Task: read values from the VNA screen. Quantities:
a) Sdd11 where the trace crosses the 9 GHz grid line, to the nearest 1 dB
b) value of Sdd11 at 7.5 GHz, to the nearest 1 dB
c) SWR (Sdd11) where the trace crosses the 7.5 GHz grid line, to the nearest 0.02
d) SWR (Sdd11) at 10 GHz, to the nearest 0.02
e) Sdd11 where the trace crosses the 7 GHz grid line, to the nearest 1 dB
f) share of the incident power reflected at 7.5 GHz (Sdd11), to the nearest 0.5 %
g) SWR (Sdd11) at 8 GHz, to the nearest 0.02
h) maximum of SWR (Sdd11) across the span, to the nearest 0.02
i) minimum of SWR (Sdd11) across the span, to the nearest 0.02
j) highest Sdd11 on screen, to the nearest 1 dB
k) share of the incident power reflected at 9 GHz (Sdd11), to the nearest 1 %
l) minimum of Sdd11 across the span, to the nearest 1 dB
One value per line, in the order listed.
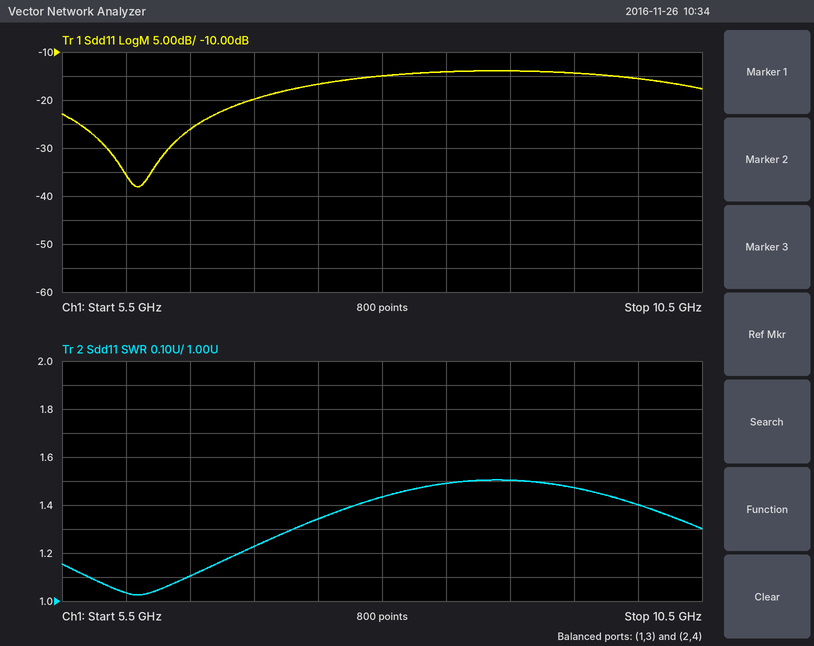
-14 dB
-17 dB
1.34
1.40
-20 dB
2.0 %
1.44
1.50
1.02
-14 dB
4 %
-38 dB
